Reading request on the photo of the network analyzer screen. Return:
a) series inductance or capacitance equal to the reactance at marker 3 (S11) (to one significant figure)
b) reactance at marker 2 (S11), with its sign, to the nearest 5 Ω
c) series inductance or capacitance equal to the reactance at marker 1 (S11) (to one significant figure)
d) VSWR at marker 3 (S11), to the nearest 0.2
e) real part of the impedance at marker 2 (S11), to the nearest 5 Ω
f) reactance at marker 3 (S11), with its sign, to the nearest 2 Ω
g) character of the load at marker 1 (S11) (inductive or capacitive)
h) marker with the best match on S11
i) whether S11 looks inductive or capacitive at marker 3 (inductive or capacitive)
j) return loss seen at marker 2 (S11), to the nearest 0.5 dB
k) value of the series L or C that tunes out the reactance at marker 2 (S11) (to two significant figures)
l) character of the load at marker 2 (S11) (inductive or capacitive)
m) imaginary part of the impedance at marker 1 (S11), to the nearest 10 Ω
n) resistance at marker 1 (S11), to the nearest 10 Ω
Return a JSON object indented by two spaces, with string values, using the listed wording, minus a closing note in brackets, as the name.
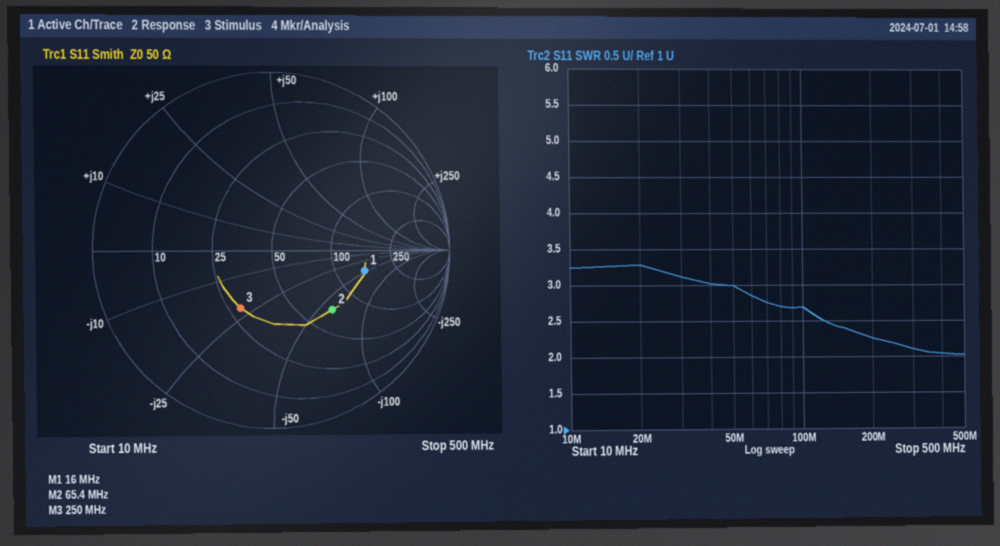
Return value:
{
  "series inductance or capacitance equal to the reactance at marker 3 (S11)": "30 pF",
  "reactance at marker 2 (S11), with its sign, to the nearest 5 Ω": "-60 Ω",
  "series inductance or capacitance equal to the reactance at marker 1 (S11)": "200 pF",
  "VSWR at marker 3 (S11), to the nearest 0.2": "2.2",
  "real part of the impedance at marker 2 (S11), to the nearest 5 Ω": "70 Ω",
  "reactance at marker 3 (S11), with its sign, to the nearest 2 Ω": "-22 Ω",
  "character of the load at marker 1 (S11)": "capacitive",
  "marker with the best match on S11": "marker 3",
  "whether S11 looks inductive or capacitive at marker 3": "capacitive",
  "return loss seen at marker 2 (S11), to the nearest 0.5 dB": "6.5 dB",
  "value of the series L or C that tunes out the reactance at marker 2 (S11)": "150 nH",
  "character of the load at marker 2 (S11)": "capacitive",
  "imaginary part of the impedance at marker 1 (S11), to the nearest 10 Ω": "-50 Ω",
  "resistance at marker 1 (S11), to the nearest 10 Ω": "150 Ω"
}
